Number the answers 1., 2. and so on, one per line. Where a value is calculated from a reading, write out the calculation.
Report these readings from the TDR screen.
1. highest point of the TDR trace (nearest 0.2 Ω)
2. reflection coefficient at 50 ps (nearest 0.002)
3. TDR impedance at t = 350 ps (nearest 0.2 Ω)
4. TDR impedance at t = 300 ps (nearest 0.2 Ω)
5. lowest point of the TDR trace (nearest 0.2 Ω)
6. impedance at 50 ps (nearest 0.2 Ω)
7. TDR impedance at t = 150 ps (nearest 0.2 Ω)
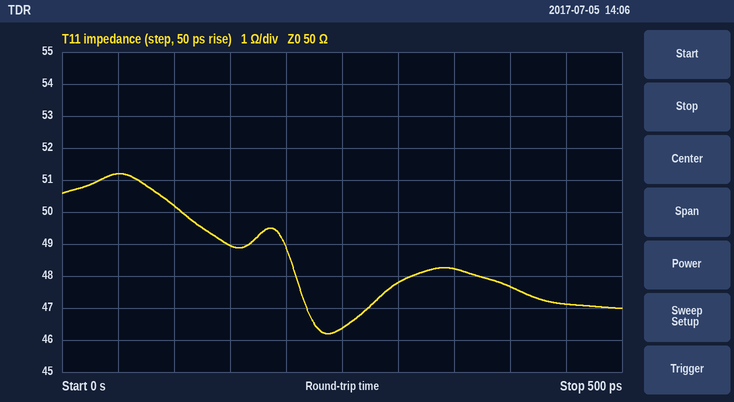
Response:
1. 51.2 Ω
2. (51.2 − 50)/(51.2 + 50) ≈ +0.012
3. 48.2 Ω
4. 47.8 Ω
5. 46.2 Ω
6. 51.2 Ω
7. 49.0 Ω
